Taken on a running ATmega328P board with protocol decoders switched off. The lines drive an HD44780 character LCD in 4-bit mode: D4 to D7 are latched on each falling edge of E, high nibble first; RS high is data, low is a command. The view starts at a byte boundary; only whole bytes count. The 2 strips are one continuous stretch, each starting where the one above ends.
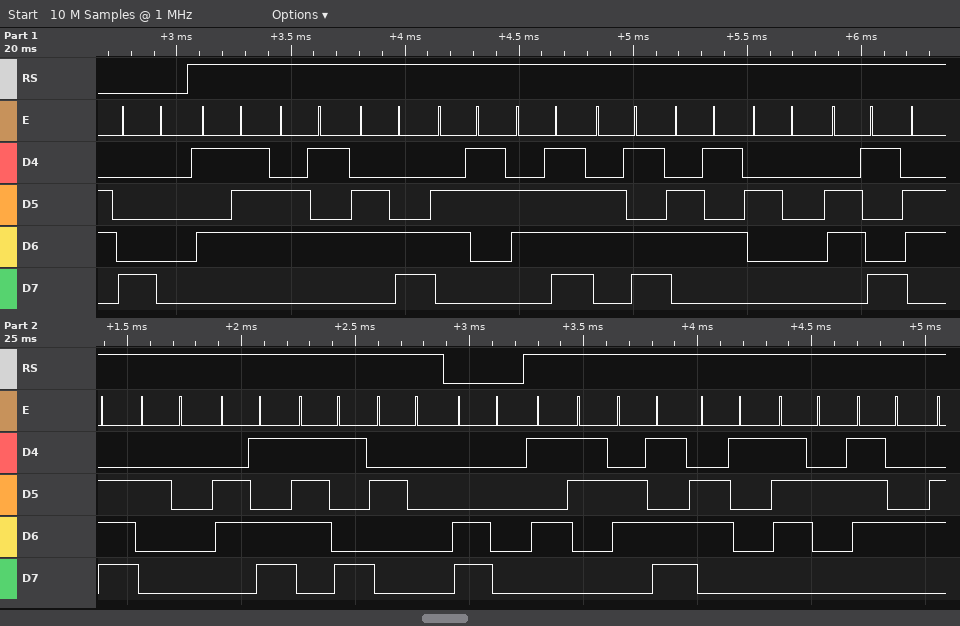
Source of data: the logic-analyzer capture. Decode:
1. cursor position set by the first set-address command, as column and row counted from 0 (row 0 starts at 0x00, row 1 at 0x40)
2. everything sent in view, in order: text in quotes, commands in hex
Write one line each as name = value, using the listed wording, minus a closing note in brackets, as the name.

cursor position set by the first set-address command, as column and row counted from 0 = column 0, row 0
everything sent in view, in order: text in quotes, commands in hex = 0x80 "Welcome in my " 0xC0 "Smart"
